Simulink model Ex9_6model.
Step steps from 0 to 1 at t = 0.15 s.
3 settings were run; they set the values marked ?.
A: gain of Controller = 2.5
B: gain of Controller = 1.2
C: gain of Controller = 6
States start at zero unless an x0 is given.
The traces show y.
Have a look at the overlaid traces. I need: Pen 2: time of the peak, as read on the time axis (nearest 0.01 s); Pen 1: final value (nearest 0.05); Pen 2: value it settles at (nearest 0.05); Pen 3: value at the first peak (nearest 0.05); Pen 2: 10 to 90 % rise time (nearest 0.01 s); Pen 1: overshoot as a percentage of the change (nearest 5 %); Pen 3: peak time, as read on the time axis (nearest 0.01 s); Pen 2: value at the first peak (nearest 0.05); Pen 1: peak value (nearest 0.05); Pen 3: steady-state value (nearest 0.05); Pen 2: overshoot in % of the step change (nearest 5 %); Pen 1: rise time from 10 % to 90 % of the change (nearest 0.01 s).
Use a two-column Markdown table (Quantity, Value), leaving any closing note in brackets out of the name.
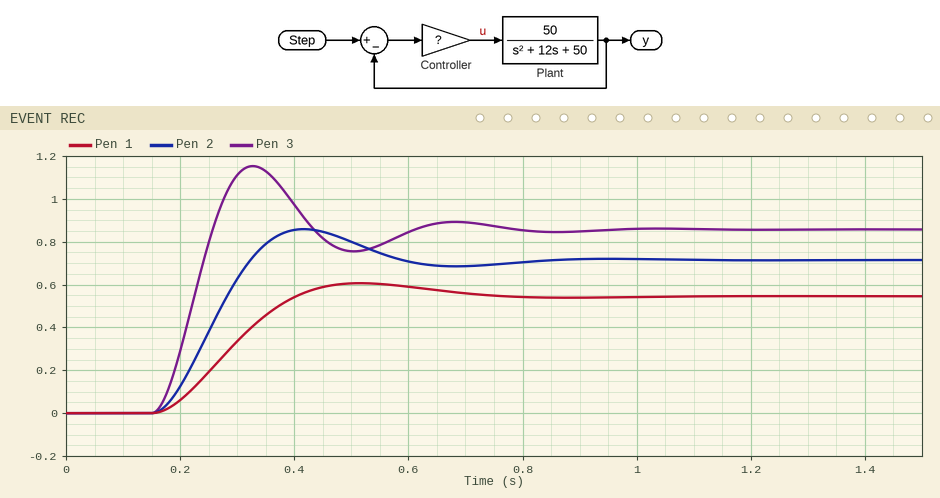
| Quantity | Value |
|---|---|
| Pen 2: time of the peak, as read on the time axis | 0.42 s |
| Pen 1: final value | 0.55 |
| Pen 2: value it settles at | 0.70 |
| Pen 3: value at the first peak | 1.15 |
| Pen 2: 10 to 90 % rise time | 0.12 s |
| Pen 1: overshoot as a percentage of the change | 10 % |
| Pen 3: peak time, as read on the time axis | 0.33 s |
| Pen 2: value at the first peak | 0.85 |
| Pen 1: peak value | 0.60 |
| Pen 3: steady-state value | 0.85 |
| Pen 2: overshoot in % of the step change | 20 % |
| Pen 1: rise time from 10 % to 90 % of the change | 0.17 s |
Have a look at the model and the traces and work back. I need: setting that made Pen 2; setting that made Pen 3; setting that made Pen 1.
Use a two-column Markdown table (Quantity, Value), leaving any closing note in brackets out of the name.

| Quantity | Value |
|---|---|
| setting that made Pen 2 | A |
| setting that made Pen 3 | C |
| setting that made Pen 1 | B |
